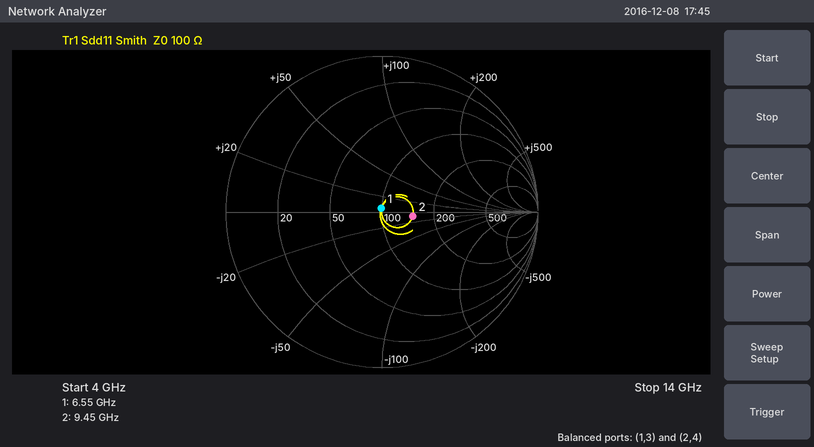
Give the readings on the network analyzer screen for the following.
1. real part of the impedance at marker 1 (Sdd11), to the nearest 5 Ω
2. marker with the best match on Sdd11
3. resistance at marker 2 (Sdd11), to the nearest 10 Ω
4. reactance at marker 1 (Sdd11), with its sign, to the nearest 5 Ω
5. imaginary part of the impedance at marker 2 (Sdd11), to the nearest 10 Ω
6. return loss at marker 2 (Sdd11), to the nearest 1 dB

100 Ω
marker 1
150 Ω
+5 Ω
-10 Ω
14 dB
